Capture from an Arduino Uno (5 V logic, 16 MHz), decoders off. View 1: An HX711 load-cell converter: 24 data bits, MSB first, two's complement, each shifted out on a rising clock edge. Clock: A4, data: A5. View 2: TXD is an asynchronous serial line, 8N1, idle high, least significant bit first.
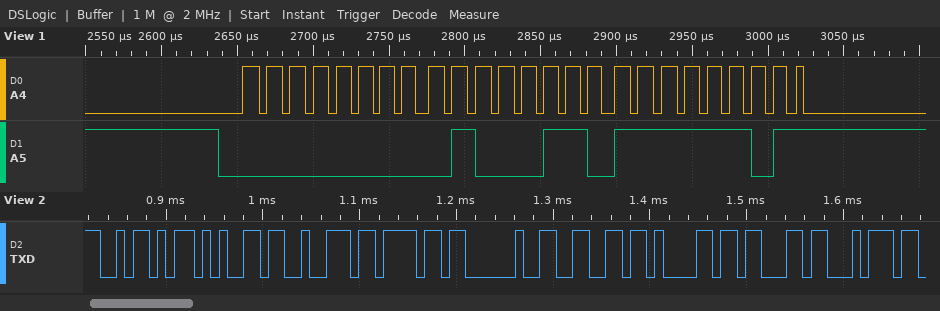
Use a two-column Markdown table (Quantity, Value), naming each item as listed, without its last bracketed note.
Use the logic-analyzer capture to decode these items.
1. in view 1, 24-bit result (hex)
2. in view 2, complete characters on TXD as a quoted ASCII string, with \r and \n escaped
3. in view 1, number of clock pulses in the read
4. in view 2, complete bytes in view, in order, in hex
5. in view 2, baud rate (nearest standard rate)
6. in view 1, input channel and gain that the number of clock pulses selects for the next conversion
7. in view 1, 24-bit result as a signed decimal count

| Quantity | Value |
|---|---|
| in view 1, 24-bit result | 0x0046FD |
| in view 2, complete characters on TXD as a quoted ASCII string, with \r and \n escaped | "Zero fact" |
| in view 1, number of clock pulses in the read | 25 |
| in view 2, complete bytes in view, in order, in hex | 5A 65 72 6F 20 66 61 63 74 |
| in view 2, baud rate | 115200 baud |
| in view 1, input channel and gain that the number of clock pulses selects for the next conversion | channel A, gain 128 |
| in view 1, 24-bit result as a signed decimal count | 18173 |
